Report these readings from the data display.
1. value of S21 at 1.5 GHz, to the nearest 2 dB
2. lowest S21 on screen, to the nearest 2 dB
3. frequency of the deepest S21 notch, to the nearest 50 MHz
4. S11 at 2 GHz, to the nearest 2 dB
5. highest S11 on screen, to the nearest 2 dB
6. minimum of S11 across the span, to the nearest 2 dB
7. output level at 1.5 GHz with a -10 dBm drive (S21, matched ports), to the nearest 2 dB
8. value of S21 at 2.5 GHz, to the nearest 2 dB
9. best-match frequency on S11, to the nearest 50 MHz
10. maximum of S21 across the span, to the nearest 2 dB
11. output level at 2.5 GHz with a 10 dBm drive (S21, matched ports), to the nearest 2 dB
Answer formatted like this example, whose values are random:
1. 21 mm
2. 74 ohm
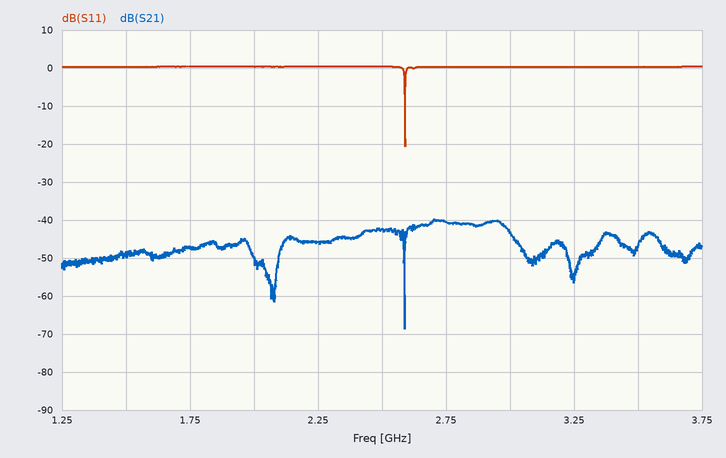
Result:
1. -48 dB
2. -68 dB
3. 2.60 GHz
4. 0 dB
5. 0 dB
6. -20 dB
7. -58 dBm
8. -42 dB
9. 2.60 GHz
10. -40 dB
11. -32 dBm
